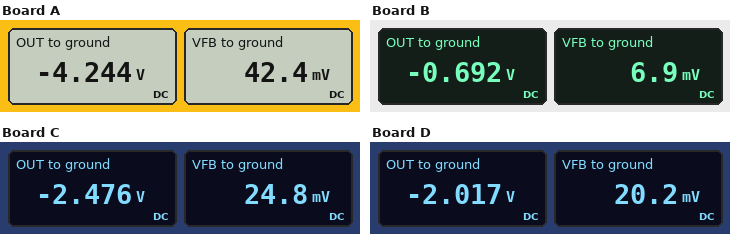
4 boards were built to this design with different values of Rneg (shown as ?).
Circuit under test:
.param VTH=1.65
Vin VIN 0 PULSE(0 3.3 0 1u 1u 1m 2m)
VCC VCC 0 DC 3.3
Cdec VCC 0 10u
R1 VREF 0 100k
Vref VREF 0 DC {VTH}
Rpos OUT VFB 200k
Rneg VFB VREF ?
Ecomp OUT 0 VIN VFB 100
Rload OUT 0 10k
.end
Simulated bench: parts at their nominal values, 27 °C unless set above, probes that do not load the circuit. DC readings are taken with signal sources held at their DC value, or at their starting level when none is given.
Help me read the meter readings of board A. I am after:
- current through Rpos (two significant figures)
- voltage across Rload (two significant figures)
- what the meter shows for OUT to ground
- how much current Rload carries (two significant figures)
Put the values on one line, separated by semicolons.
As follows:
21 µA; 4.2 V; -4.244 V; 420 µA
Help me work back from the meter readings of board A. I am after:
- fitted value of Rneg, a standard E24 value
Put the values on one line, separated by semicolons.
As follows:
75 kΩ
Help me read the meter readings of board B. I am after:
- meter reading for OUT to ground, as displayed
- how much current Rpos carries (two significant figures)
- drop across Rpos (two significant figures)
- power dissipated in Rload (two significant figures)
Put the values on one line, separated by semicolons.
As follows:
-0.692 V; 3.5 µA; 700 mV; 48 µW
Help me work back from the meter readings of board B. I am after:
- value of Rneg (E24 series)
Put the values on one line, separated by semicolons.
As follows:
470 kΩ
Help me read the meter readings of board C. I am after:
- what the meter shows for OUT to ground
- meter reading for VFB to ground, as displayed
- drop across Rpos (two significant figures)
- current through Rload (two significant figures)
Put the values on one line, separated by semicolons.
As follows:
-2.476 V; 24.8 mV; 2.5 V; 250 µA
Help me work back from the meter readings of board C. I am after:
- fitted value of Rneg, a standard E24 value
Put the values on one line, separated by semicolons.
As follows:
130 kΩ
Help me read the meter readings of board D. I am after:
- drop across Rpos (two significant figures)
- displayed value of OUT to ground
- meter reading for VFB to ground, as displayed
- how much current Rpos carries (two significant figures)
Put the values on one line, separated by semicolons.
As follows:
2.0 V; -2.017 V; 20.2 mV; 10 µA
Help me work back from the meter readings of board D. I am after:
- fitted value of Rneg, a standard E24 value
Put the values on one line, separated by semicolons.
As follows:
160 kΩ
